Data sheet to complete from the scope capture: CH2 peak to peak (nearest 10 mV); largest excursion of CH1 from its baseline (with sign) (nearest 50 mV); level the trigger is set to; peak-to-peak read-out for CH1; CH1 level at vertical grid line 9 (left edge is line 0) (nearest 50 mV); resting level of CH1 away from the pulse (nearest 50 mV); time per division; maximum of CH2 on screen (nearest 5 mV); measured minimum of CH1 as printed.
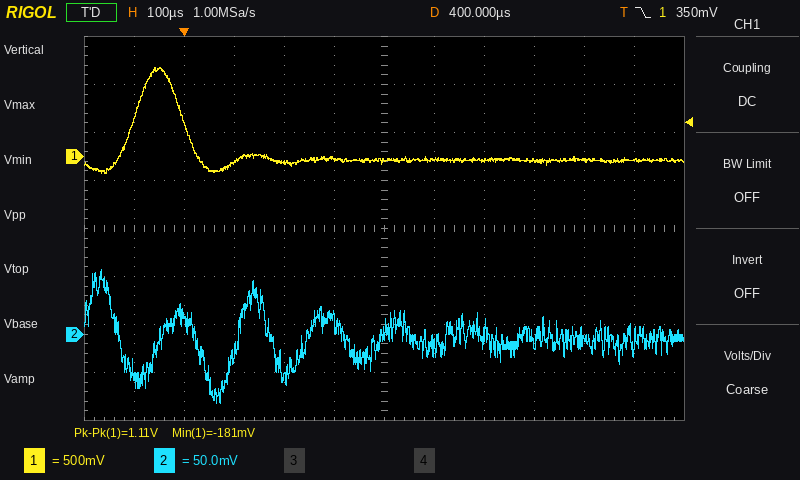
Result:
140 mV
+950 mV
350 mV
1.11 V
-50 mV
-50 mV
100 µs
65 mV
-181 mV
